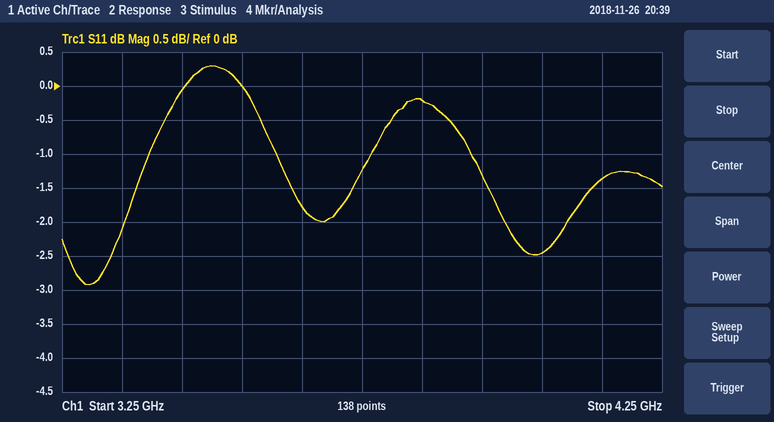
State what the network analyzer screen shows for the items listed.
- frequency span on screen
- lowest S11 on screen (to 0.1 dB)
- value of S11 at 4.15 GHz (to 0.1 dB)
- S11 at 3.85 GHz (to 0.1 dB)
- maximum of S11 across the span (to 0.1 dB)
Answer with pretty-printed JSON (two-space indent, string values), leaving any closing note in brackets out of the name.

{
  "frequency span on screen": "1 GHz",
  "lowest S11 on screen": "-2.9 dB",
  "value of S11 at 4.15 GHz": "-1.4 dB",
  "S11 at 3.85 GHz": "-0.2 dB",
  "maximum of S11 across the span": "0.3 dB"
}
